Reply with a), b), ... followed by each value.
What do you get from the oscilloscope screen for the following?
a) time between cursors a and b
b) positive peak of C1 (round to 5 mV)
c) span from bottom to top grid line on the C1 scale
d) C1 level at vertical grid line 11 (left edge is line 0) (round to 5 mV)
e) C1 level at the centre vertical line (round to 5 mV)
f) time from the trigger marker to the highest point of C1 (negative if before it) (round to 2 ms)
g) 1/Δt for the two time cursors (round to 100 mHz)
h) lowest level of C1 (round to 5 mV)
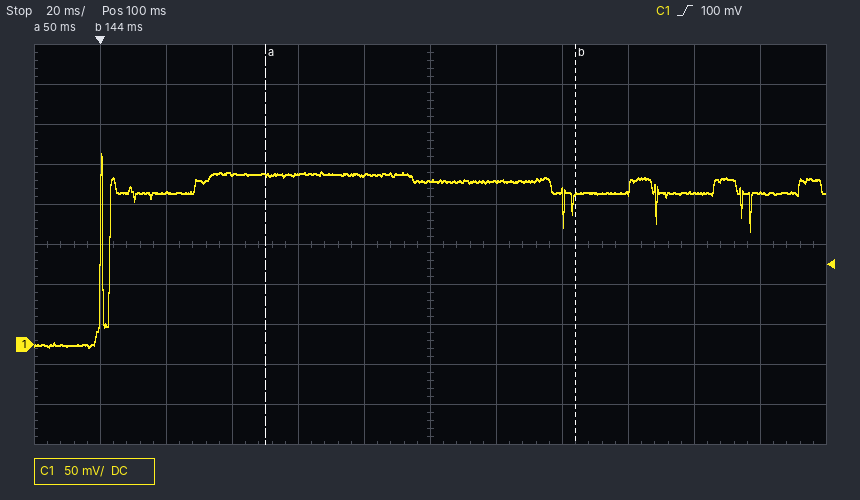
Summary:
a) 94 ms
b) 240 mV
c) 500 mV
d) 190 mV
e) 205 mV
f) 0 ms
g) 10.6 Hz
h) -5 mV
